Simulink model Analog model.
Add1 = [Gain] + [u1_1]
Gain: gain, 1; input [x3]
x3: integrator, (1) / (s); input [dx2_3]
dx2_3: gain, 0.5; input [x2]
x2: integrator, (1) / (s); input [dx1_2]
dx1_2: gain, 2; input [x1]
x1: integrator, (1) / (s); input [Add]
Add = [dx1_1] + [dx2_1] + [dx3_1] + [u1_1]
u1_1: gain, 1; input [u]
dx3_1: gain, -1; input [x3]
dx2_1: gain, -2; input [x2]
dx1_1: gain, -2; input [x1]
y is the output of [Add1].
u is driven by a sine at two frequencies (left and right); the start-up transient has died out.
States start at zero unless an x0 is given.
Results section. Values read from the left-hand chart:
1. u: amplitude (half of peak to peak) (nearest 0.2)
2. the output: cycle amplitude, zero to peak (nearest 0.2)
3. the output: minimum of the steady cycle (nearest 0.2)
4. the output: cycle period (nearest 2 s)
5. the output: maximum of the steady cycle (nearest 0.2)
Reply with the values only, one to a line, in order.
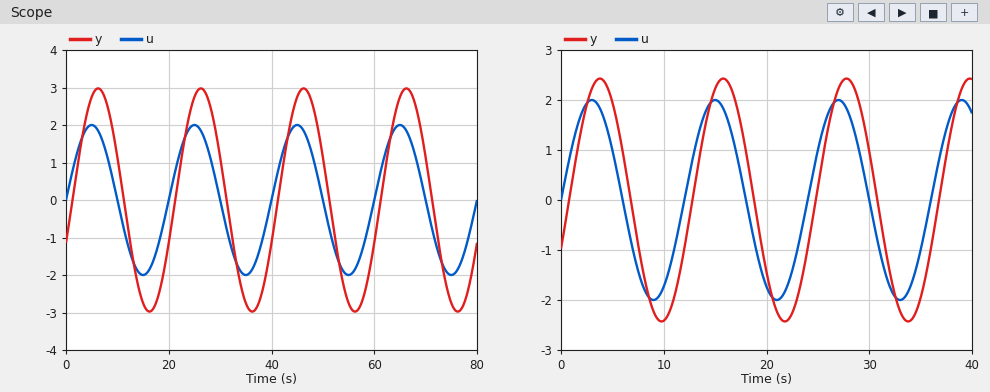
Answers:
2.0
3.0
-3.0
20 s
3.0
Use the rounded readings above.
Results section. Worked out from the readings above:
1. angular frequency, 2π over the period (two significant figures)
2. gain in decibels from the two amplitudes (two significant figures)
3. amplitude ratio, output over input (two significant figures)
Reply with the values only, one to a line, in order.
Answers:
0.31 rad/s
3.5 dB
1.5
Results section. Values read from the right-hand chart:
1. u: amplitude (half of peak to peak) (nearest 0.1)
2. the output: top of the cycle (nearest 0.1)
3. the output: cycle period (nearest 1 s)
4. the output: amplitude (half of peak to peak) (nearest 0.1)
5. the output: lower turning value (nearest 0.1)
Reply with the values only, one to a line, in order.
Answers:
2.0
2.4
12 s
2.4
-2.4
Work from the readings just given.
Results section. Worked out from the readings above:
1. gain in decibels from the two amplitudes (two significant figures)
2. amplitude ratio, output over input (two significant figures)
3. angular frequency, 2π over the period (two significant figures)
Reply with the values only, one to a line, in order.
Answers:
1.6 dB
1.2
0.52 rad/s
